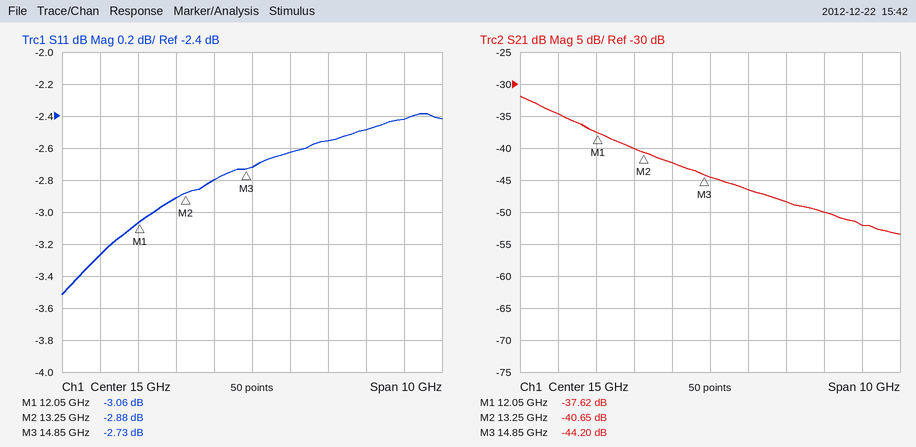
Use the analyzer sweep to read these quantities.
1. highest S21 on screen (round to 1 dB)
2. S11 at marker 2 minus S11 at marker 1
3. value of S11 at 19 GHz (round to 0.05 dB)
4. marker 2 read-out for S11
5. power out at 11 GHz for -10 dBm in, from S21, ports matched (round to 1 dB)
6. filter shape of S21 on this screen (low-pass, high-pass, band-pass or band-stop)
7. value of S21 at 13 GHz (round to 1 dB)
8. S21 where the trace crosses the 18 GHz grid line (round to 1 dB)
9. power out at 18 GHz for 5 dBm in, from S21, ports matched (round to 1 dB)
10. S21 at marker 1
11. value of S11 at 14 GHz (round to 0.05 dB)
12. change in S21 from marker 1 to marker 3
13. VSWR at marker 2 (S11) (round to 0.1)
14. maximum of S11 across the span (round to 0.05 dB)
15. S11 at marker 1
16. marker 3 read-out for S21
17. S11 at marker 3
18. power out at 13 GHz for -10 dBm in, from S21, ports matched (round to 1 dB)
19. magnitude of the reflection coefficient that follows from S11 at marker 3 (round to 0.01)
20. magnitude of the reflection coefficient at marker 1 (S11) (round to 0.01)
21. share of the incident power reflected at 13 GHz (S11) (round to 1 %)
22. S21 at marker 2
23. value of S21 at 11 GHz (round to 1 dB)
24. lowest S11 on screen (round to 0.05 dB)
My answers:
-32 dB
0.18 dB
-2.40 dB
-2.88 dB
-45 dBm
low-pass
-40 dB
-50 dB
-45 dBm
-37.62 dB
-2.80 dB
-6.58 dB
6.1
-2.40 dB
-3.06 dB
-44.20 dB
-2.73 dB
-50 dBm
0.73
0.70
51 %
-40.65 dB
-35 dB
-3.50 dB
